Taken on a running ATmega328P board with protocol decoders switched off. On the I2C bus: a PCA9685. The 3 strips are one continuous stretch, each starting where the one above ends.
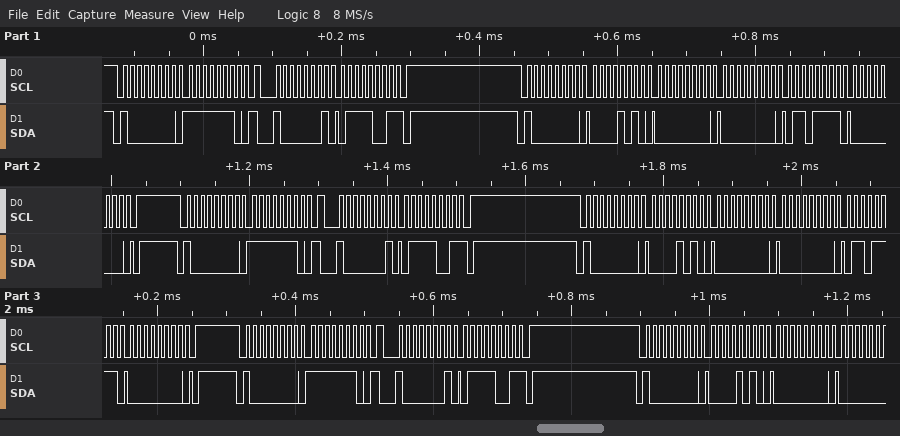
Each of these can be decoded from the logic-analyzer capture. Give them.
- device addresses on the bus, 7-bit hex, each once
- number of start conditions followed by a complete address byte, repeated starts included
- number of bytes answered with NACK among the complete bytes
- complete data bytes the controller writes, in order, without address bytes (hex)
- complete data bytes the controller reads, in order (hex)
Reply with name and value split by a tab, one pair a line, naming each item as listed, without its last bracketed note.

device addresses on the bus, 7-bit hex, each once	0x40
number of start conditions followed by a complete address byte, repeated starts included	9
number of bytes answered with NACK among the complete bytes	3
complete data bytes the controller writes, in order, without address bytes	FE 0A 00 00 6F 00 FE 0A 00 00 6F 00 FE 0A 00
complete data bytes the controller reads, in order	79 79 79
